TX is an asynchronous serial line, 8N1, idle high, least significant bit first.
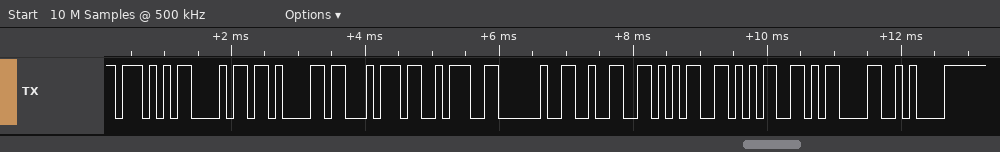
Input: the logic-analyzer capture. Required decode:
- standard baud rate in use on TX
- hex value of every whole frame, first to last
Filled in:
9600 baud
0x57 0x68 0x61 0x74 0x3A 0x20 0x32 0x35 0x35 0x0D 0x0A
